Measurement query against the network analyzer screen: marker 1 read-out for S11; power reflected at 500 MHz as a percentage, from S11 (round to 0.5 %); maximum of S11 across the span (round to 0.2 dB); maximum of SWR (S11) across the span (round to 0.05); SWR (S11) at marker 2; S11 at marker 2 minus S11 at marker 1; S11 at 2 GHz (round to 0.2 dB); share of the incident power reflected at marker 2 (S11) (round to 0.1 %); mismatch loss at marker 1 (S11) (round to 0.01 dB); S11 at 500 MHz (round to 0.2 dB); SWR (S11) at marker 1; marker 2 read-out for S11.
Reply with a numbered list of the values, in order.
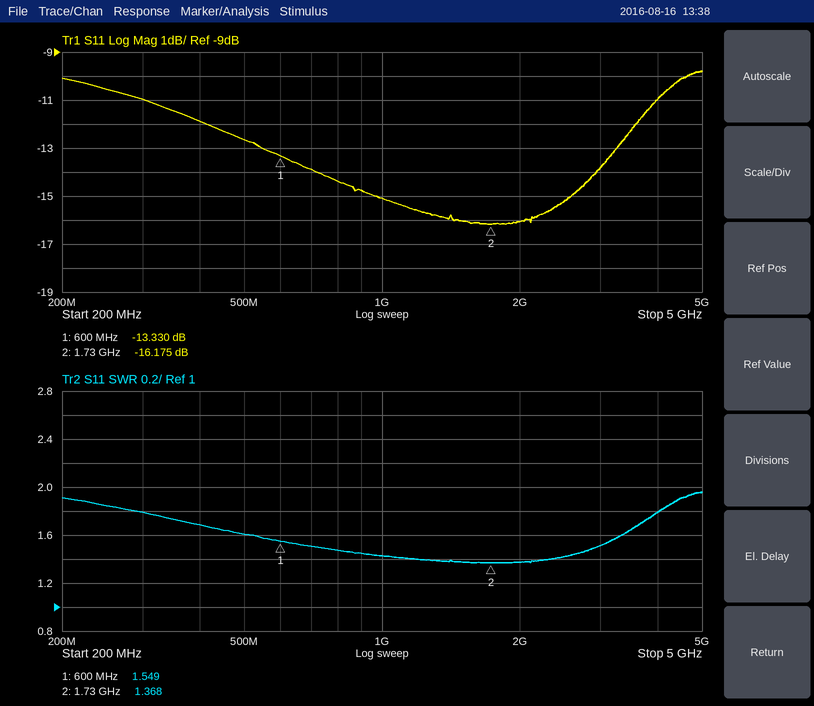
1. -13.330 dB
2. 5.5 %
3. -9.8 dB
4. 1.95
5. 1.368
6. -2.845 dB
7. -16.0 dB
8. 2.4 %
9. 0.21 dB
10. -12.6 dB
11. 1.549
12. -16.175 dB
